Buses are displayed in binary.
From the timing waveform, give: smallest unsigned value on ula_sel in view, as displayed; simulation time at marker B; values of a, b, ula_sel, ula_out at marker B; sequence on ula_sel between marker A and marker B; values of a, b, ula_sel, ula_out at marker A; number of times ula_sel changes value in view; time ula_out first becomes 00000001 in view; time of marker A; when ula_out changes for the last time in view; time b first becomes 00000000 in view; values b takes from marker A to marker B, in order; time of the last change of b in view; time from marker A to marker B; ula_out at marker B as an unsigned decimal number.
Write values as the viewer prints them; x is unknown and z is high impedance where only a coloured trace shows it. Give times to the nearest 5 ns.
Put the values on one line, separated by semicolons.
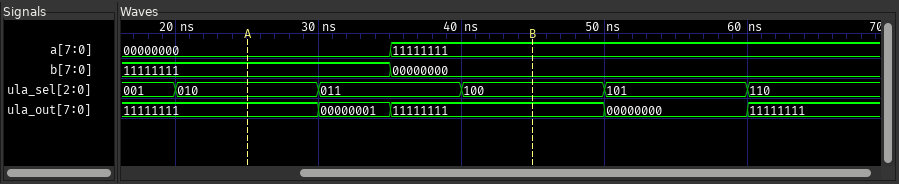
001; 45 ns; a=11111111, b=00000000, ula_sel=100, ula_out=11111111; 010, 011, 100; a=00000000, b=11111111, ula_sel=010, ula_out=11111111; 5; 30 ns; 25 ns; 60 ns; 35 ns; 11111111, 00000000; 35 ns; 20 ns; 255
